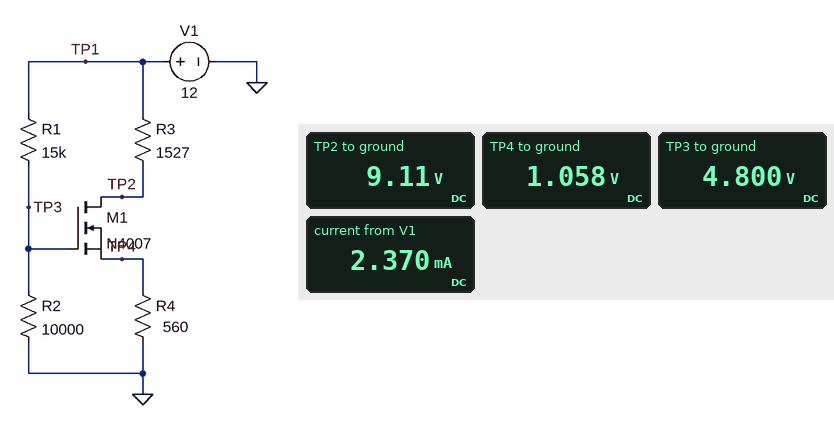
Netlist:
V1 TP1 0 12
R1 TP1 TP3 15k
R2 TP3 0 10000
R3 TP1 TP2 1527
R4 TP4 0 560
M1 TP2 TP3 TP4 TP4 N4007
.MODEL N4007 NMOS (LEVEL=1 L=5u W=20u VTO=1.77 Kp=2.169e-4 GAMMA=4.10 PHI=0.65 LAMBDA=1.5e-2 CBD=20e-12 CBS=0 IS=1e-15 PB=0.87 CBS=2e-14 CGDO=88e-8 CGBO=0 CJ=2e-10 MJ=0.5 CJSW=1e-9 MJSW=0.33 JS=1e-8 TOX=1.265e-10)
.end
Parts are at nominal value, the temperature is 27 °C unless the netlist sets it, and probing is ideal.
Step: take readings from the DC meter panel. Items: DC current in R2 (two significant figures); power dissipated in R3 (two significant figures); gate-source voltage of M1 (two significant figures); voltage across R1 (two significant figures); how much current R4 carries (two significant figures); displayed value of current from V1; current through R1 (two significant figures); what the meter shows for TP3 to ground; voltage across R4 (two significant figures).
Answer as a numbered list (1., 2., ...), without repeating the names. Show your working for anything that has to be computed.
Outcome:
1. (4.8 V) / 10 kΩ = 480 µA
2. (12 V - 9.11 V)^2 / 1.527 kΩ = 5.5 mW
3. 4.8 V - 1.058 V = 3.7 V
4. 12 V - 4.8 V = 7.2 V
5. (1.058 V) / 560 Ω = 1.9 mA
6. 2.370 mA
7. (12 V - 4.8 V) / 15 kΩ = 480 µA
8. 4.800 V
9. 1.058 V = 1.1 V
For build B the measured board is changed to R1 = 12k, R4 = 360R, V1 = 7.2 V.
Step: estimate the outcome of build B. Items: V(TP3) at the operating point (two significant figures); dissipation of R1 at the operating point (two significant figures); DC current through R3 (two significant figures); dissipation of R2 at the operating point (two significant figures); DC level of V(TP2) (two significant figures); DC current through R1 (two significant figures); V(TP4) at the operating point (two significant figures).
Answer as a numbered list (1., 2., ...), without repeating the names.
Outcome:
1. 3.3 V
2. 1.3 mW
3. 730 µA
4. 1.1 mW
5. 6.1 V
6. 330 µA
7. 260 mV
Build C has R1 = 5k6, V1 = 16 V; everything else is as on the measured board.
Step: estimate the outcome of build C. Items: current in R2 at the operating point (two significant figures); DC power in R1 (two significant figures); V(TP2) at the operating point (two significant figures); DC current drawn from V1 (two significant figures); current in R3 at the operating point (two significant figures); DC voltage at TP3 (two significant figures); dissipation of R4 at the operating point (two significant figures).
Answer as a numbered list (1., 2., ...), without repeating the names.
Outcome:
1. 1.0 mA
2. 5.9 mW
3. 5.8 V
4. 7.7 mA
5. 6.7 mA
6. 10 V
7. 25 mW
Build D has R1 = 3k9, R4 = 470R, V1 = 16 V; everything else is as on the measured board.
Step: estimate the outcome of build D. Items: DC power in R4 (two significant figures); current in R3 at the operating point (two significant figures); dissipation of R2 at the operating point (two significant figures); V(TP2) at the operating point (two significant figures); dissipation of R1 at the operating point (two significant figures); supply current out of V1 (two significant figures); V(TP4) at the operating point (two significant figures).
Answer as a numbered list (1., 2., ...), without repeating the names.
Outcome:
1. 25 mW
2. 7.3 mA
3. 13 mW
4. 4.9 V
5. 5.2 mW
6. 8.4 mA
7. 3.4 V
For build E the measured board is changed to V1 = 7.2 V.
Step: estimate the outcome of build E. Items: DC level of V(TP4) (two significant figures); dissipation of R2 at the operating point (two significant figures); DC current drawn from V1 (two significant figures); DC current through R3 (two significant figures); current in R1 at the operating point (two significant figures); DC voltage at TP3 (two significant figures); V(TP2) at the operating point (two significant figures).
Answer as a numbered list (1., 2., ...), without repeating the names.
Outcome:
1. 210 mV
2. 830 µW
3. 670 µA
4. 380 µA
5. 290 µA
6. 2.9 V
7. 6.6 V
